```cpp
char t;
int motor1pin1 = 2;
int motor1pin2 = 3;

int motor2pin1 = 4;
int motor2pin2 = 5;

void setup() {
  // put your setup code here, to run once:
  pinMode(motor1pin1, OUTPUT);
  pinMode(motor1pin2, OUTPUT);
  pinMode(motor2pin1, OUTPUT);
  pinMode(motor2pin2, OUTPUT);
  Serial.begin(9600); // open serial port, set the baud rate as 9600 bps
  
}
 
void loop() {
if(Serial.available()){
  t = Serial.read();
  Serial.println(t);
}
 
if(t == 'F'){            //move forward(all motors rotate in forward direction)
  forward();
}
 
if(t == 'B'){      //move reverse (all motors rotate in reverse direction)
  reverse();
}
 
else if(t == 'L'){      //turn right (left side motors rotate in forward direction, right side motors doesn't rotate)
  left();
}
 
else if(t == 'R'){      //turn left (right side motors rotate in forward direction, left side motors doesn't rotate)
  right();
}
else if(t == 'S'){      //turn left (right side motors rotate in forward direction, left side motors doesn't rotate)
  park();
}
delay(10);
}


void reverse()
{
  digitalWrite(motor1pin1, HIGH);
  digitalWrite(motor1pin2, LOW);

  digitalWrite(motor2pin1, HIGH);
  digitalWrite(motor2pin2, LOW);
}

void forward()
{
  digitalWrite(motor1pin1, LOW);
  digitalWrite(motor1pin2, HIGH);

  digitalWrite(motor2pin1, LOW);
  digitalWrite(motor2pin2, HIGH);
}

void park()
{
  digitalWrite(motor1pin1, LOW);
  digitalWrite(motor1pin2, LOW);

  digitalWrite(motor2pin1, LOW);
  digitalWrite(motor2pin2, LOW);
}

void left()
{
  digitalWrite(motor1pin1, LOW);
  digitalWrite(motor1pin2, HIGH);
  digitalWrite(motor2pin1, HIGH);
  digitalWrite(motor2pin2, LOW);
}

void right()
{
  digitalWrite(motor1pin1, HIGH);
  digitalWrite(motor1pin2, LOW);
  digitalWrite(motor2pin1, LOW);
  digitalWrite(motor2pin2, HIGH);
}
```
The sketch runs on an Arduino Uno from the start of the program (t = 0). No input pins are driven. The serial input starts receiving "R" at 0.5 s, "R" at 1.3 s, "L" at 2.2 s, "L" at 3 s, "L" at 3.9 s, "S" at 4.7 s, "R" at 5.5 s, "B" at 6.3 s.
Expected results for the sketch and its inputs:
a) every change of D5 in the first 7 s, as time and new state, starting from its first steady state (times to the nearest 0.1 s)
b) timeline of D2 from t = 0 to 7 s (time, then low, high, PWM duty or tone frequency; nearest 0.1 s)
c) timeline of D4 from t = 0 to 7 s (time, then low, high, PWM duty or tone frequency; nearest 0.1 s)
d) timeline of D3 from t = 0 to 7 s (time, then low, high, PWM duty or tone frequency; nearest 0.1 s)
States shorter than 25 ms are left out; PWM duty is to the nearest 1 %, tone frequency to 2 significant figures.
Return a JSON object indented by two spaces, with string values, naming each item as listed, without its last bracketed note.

{
  "every change of D5 in the first 7 s, as time and new state, starting from its first steady state": "0 s low; 0.5 s high; 2.2 s low; 5.5 s high; 6.3 s low",
  "timeline of D2 from t = 0 to 7 s": "0 s low; 0.5 s high; 2.2 s low; 5.5 s high",
  "timeline of D4 from t = 0 to 7 s": "0 s low; 2.2 s high; 4.7 s low; 6.3 s high",
  "timeline of D3 from t = 0 to 7 s": "0 s low; 2.2 s high; 4.7 s low"
}
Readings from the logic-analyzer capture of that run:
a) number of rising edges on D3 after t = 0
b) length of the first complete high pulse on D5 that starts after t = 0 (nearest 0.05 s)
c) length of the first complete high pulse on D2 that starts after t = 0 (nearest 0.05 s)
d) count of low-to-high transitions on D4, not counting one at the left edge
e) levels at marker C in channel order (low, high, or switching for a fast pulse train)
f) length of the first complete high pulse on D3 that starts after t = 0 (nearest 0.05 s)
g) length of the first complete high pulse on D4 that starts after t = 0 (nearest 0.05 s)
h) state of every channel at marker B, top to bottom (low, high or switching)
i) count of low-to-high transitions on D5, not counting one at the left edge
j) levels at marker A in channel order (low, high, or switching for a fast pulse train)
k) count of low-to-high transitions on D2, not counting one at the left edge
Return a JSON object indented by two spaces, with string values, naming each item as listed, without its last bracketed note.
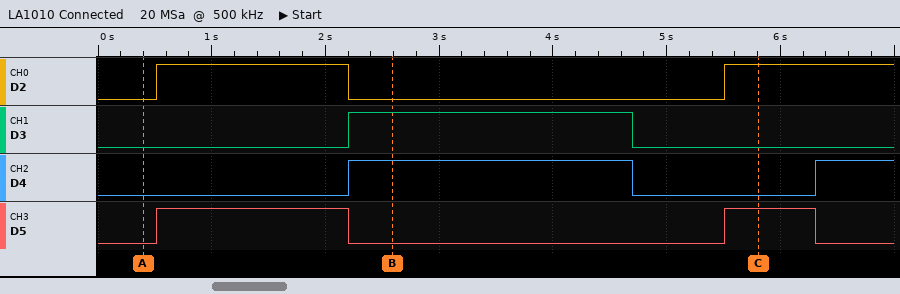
{
  "number of rising edges on D3 after t = 0": "1",
  "length of the first complete high pulse on D5 that starts after t = 0": "1.70 s",
  "length of the first complete high pulse on D2 that starts after t = 0": "1.70 s",
  "count of low-to-high transitions on D4, not counting one at the left edge": "2",
  "levels at marker C in channel order": "D2 high, D3 low, D4 low, D5 high",
  "length of the first complete high pulse on D3 that starts after t = 0": "2.50 s",
  "length of the first complete high pulse on D4 that starts after t = 0": "2.50 s",
  "state of every channel at marker B, top to bottom": "D2 low, D3 high, D4 high, D5 low",
  "count of low-to-high transitions on D5, not counting one at the left edge": "2",
  "levels at marker A in channel order": "D2 low, D3 low, D4 low, D5 low",
  "count of low-to-high transitions on D2, not counting one at the left edge": "2"
}
